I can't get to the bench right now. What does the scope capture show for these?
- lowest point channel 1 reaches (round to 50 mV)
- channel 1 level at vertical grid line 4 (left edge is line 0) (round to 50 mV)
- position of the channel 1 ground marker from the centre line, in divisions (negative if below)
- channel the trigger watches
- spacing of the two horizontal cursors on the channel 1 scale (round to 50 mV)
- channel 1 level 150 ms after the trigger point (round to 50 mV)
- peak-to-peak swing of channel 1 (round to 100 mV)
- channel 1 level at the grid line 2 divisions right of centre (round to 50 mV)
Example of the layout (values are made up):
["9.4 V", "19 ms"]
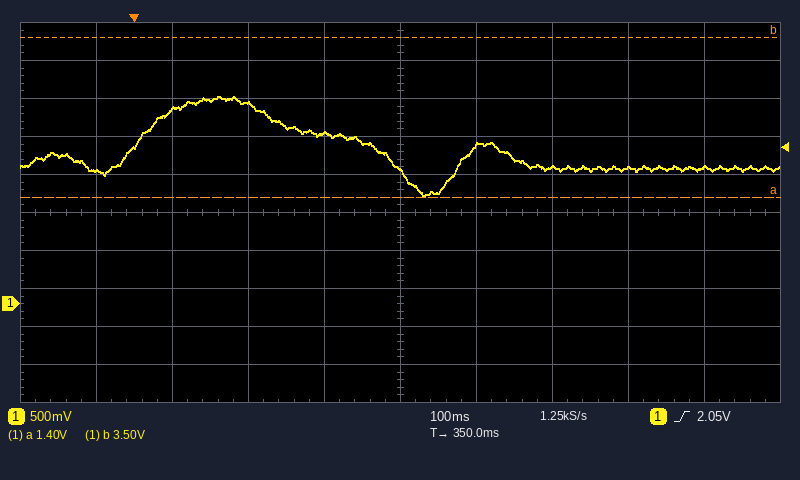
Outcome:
["1.40 V", "2.25 V", "-2.4 div", "channel 1", "2.10 V", "2.65 V", "1.30 V", "1.80 V"]
